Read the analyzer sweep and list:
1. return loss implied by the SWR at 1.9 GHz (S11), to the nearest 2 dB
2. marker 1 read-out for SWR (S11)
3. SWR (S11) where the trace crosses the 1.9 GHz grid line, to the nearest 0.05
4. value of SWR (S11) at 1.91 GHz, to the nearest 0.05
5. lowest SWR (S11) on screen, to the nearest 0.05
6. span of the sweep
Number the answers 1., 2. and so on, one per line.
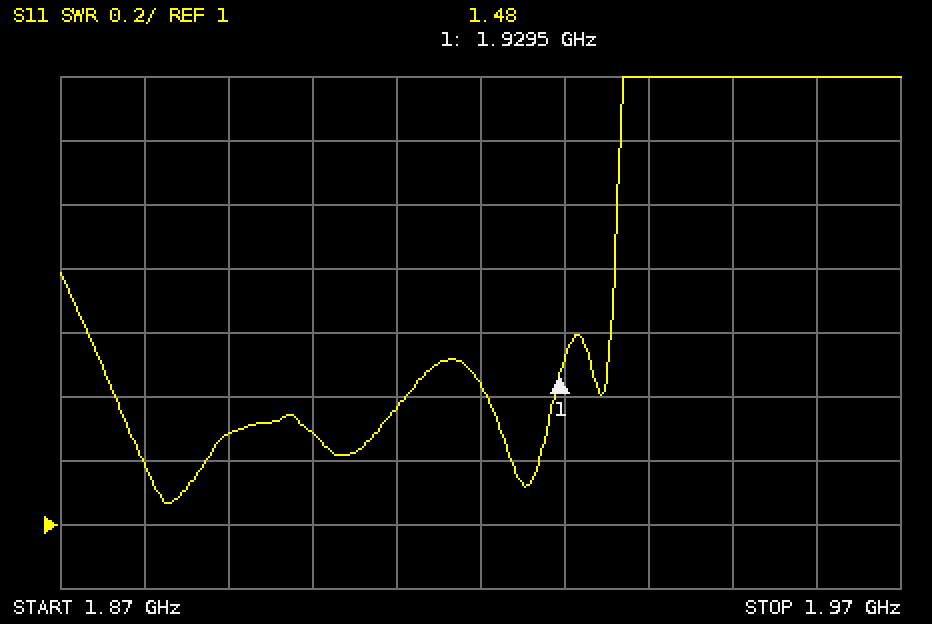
1. 18 dB
2. 1.48
3. 1.30
4. 1.35
5. 1.05
6. 100 MHz
